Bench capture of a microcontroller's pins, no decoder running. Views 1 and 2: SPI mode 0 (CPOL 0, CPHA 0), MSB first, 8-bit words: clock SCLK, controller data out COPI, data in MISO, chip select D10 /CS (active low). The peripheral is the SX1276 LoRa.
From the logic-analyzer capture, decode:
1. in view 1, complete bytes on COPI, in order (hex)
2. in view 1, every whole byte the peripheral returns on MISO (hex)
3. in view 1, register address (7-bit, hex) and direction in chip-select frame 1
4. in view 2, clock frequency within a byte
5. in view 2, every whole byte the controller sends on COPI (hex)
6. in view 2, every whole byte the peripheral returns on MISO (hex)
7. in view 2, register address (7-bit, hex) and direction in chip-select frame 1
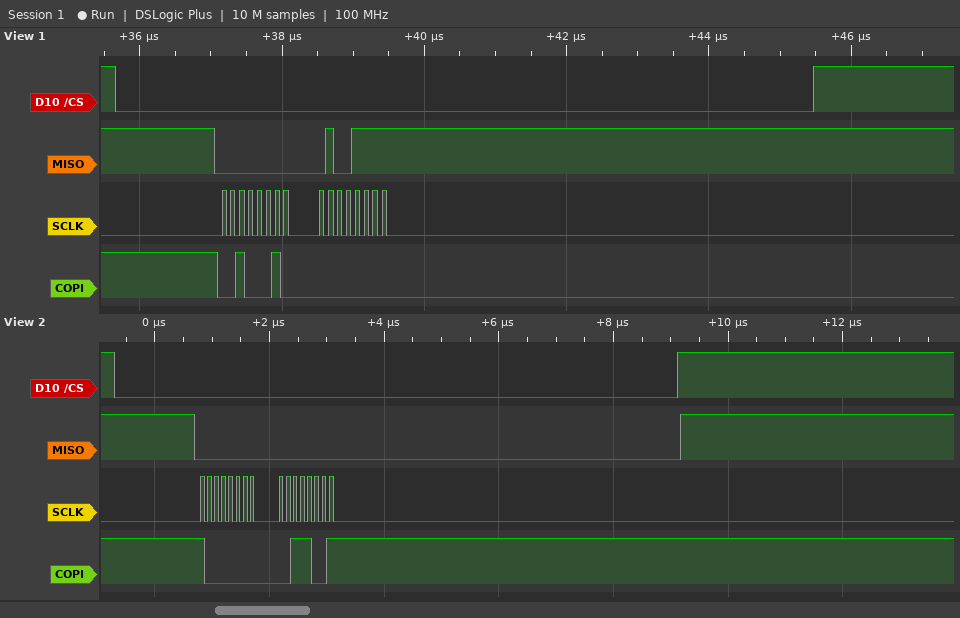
22 00
00 4F
0x22 read
8 MHz
0x80 0x39
0x00 0x00
0x00 write
